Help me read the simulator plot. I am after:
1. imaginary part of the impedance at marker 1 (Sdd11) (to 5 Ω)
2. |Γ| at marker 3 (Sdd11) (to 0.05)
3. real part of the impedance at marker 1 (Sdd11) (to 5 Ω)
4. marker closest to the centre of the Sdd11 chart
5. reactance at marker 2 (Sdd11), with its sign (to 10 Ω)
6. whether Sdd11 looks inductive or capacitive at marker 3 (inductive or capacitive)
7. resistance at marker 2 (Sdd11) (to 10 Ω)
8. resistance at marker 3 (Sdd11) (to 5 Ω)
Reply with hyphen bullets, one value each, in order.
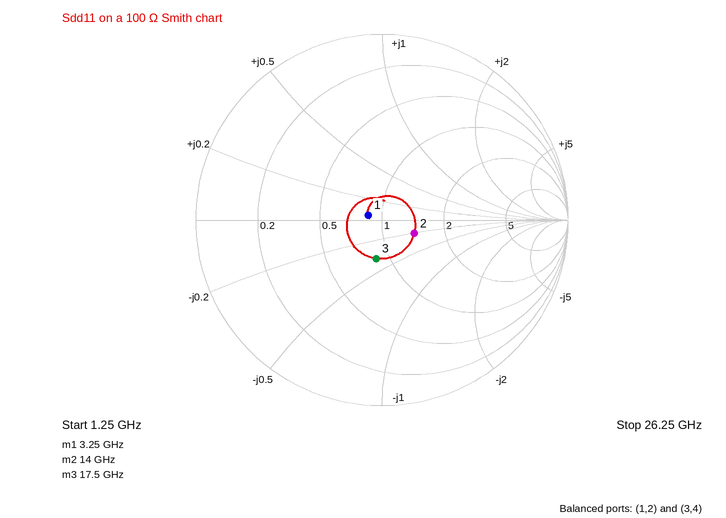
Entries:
- +5 Ω
- 0.20
- 85 Ω
- marker 1
- -20 Ω
- capacitive
- 140 Ω
- 85 Ω
